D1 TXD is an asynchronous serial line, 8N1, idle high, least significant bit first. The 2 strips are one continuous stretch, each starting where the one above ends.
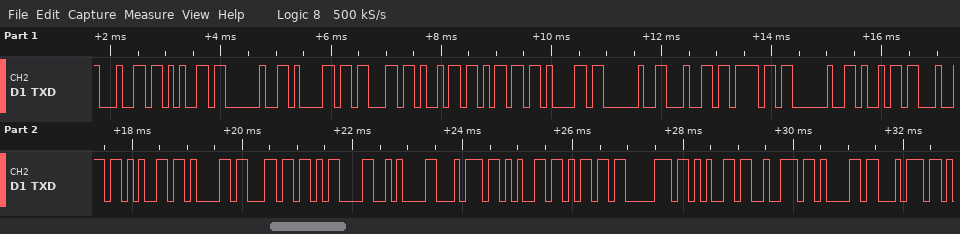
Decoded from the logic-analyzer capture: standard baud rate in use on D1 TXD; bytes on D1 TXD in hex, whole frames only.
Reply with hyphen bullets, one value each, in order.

- 9600 baud
- 64 65 20 61 63 69 6D 61 20 64 6F 20 69 64 65 61 6C 0D 0A 74 65 6D 70 65 72 61 74
